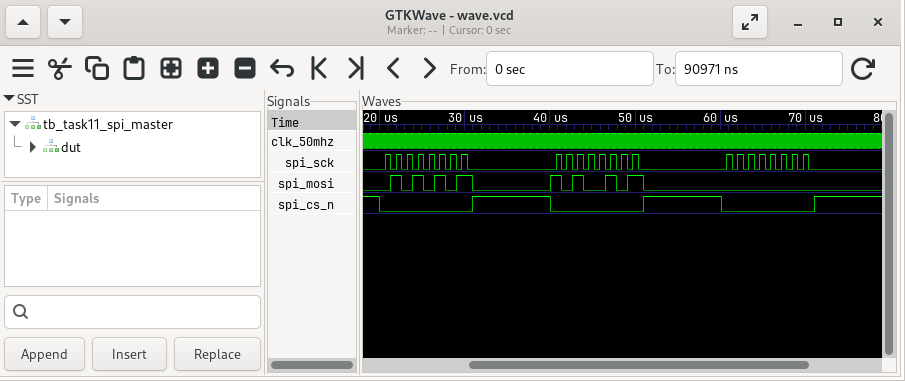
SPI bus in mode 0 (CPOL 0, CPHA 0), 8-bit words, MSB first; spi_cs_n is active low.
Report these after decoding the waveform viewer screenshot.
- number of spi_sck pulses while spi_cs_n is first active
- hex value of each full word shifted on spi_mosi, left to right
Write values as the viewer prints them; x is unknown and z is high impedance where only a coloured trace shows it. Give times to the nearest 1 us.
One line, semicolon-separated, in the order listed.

8; 55, A5, 00
